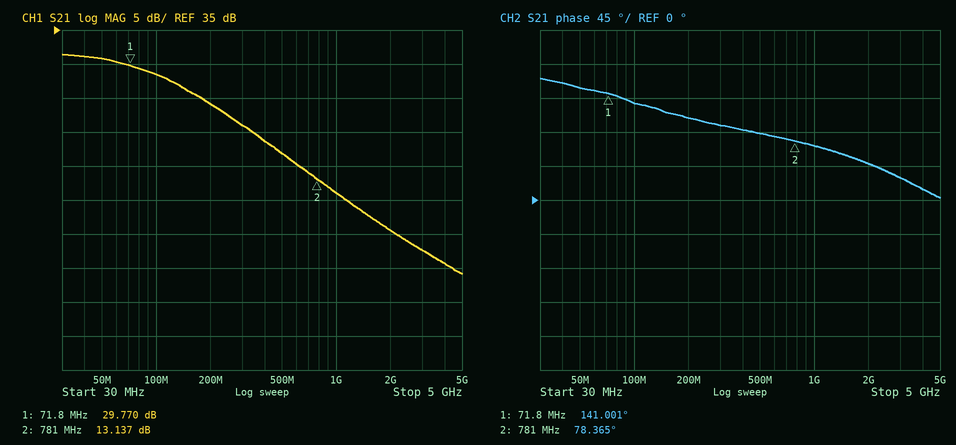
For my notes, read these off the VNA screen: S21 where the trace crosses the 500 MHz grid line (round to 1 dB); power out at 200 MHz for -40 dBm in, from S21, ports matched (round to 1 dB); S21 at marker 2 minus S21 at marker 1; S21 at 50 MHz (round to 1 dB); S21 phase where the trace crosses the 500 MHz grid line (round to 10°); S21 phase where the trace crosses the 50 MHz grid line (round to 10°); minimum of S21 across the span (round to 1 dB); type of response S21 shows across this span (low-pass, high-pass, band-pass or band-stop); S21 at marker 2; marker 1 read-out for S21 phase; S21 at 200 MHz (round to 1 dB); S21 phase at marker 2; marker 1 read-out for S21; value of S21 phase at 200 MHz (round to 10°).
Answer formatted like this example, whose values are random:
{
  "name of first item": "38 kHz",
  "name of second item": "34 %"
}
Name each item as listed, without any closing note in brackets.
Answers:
{
  "S21 where the trace crosses the 500 MHz grid line": "17 dB",
  "power out at 200 MHz for -40 dBm in, from S21, ports matched": "-16 dBm",
  "S21 at marker 2 minus S21 at marker 1": "-16.633 dB",
  "S21 at 50 MHz": "31 dB",
  "S21 phase where the trace crosses the 500 MHz grid line": "90°",
  "S21 phase where the trace crosses the 50 MHz grid line": "150°",
  "minimum of S21 across the span": "-1 dB",
  "type of response S21 shows across this span": "low-pass",
  "S21 at marker 2": "13.137 dB",
  "marker 1 read-out for S21 phase": "141.001°",
  "S21 at 200 MHz": "24 dB",
  "S21 phase at marker 2": "78.365°",
  "marker 1 read-out for S21": "29.770 dB",
  "value of S21 phase at 200 MHz": "110°"
}
